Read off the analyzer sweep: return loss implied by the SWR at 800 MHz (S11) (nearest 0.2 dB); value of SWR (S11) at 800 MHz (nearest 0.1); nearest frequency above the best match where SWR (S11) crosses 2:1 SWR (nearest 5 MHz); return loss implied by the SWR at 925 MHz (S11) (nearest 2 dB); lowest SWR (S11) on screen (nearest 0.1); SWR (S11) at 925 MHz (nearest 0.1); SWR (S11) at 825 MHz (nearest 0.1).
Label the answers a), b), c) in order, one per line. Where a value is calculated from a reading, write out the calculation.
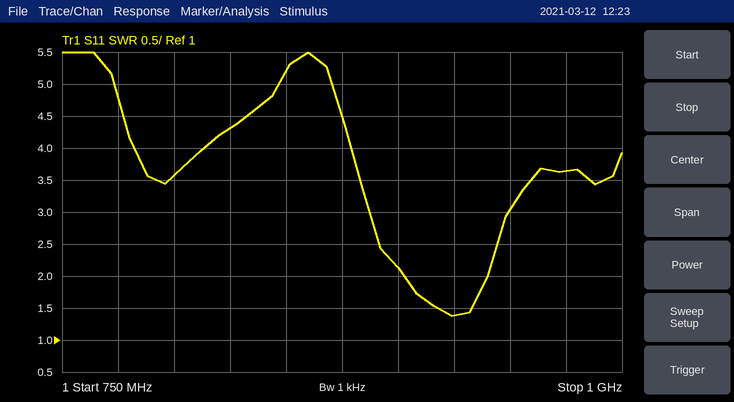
a) −20 log10((3.6 − 1)/(3.6 + 1)) ≈ 5.0 dB
b) 3.6
c) 940 MHz
d) −20 log10((1.4 − 1)/(1.4 + 1)) ≈ 16 dB
e) 1.4
f) 1.4
g) 4.3
